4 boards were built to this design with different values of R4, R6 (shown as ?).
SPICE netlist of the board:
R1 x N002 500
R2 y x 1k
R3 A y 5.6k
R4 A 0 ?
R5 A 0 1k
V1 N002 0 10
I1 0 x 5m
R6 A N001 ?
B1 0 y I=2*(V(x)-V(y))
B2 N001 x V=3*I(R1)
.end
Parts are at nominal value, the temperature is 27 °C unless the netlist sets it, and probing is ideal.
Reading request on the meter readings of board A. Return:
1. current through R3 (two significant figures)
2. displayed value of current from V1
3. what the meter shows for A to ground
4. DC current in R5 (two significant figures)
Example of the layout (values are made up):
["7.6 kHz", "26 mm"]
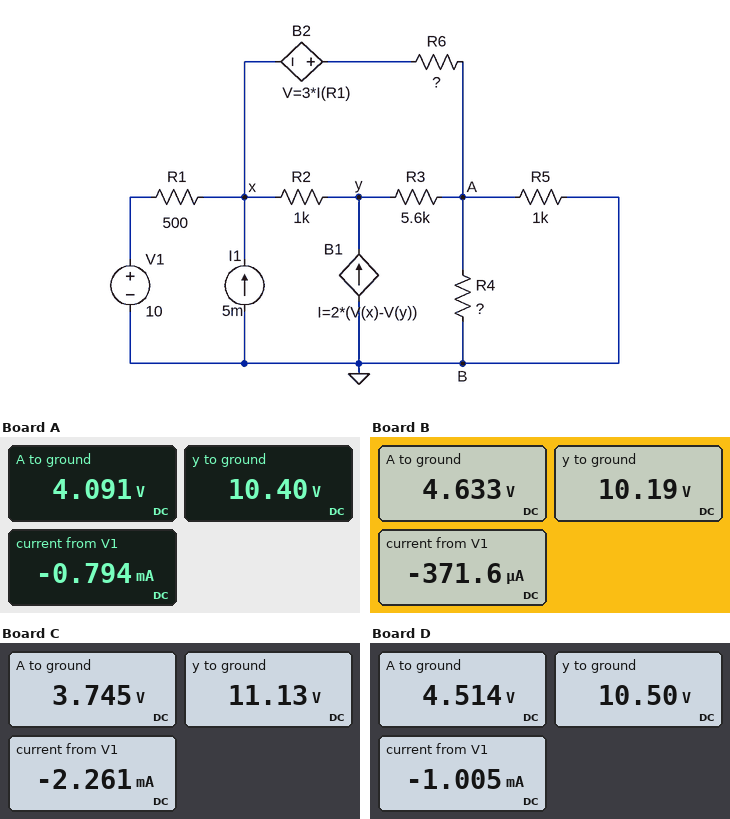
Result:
["1.1 mA", "-0.794 mA", "4.091 V", "4.1 mA"]
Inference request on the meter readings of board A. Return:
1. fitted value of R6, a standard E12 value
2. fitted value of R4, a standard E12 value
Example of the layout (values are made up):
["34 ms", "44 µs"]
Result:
["1.5 kΩ", "3.3 kΩ"]
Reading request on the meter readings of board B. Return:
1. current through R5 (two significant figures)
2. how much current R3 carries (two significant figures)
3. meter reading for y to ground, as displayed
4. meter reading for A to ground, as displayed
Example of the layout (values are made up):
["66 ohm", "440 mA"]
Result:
["4.6 mA", "990 µA", "10.19 V", "4.633 V"]
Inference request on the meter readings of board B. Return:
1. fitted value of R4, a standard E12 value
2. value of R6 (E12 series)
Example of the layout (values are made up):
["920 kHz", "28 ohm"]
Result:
["4.7 kΩ", "1.2 kΩ"]
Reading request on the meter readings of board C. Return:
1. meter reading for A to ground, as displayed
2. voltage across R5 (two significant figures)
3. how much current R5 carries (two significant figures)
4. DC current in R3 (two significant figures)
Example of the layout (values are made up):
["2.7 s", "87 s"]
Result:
["3.745 V", "3.7 V", "3.7 mA", "1.3 mA"]
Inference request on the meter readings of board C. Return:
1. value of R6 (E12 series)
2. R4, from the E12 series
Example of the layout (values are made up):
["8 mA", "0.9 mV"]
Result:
["2.7 kΩ", "12 kΩ"]
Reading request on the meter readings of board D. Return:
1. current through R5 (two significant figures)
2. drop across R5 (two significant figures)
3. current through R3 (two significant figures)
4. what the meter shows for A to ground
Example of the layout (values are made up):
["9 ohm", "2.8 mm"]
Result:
["4.5 mA", "4.5 V", "1.1 mA", "4.514 V"]
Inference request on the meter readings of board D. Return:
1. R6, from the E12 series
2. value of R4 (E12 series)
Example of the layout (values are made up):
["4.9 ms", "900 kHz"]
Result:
["1.5 kΩ", "8.2 kΩ"]
